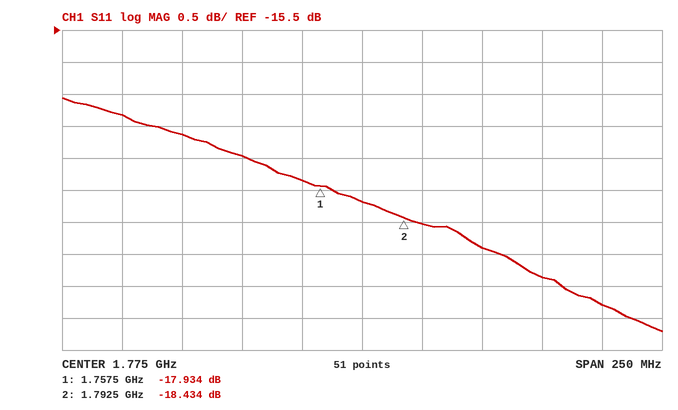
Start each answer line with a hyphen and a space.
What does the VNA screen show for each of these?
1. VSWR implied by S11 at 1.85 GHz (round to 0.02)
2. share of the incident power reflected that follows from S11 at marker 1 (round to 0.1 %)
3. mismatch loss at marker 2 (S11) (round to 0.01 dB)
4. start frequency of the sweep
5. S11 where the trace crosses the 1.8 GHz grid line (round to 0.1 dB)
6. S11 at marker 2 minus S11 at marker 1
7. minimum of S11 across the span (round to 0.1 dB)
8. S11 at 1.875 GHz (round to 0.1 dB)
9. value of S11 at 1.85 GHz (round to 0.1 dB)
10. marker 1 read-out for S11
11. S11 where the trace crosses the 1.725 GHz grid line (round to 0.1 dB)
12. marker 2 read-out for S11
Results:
- 1.24
- 1.6 %
- 0.06 dB
- 1.65 GHz
- -18.5 dB
- -0.500 dB
- -20.2 dB
- -19.8 dB
- -19.4 dB
- -17.934 dB
- -17.5 dB
- -18.434 dB
